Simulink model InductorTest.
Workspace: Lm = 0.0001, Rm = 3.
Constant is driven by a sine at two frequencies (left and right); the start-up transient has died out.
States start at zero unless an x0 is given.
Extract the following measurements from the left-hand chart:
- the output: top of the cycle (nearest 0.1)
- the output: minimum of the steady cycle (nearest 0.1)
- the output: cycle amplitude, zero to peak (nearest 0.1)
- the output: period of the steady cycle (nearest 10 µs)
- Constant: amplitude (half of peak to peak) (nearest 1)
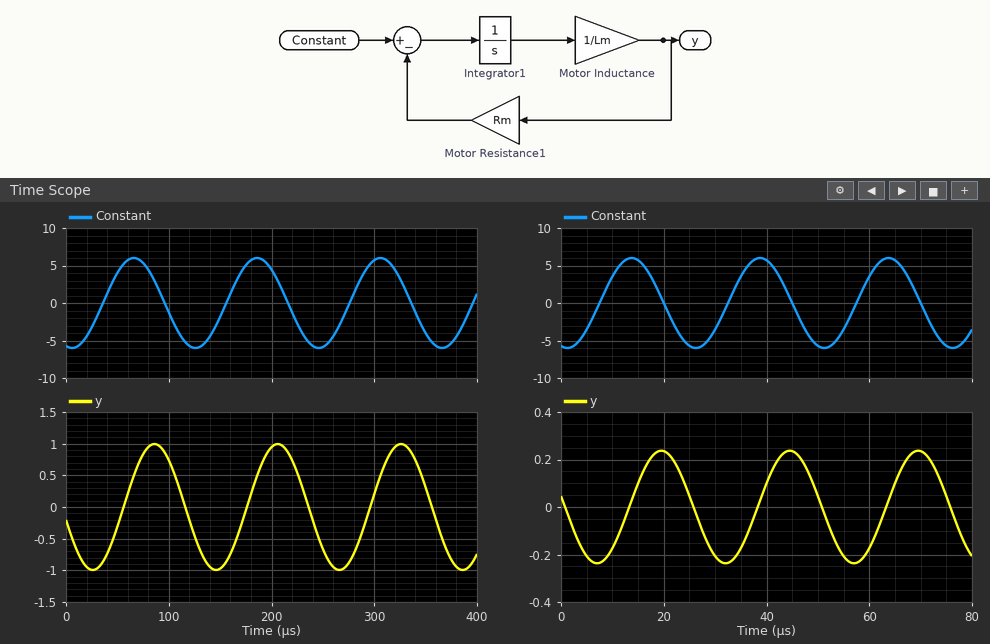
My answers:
1.0
-1.0
1.0
120 µs
6
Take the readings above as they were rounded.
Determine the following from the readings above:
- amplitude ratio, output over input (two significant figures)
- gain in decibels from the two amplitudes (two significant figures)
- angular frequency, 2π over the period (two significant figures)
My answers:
0.17
-16 dB
0.052 rad/µs
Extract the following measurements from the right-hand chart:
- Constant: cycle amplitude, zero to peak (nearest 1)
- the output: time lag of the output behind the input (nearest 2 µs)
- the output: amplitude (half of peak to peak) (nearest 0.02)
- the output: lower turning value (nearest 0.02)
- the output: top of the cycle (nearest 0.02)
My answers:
6
6 µs
0.24
-0.24
0.24
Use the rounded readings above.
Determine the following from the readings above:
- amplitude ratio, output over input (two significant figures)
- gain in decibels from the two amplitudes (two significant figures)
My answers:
0.040
-28 dB
